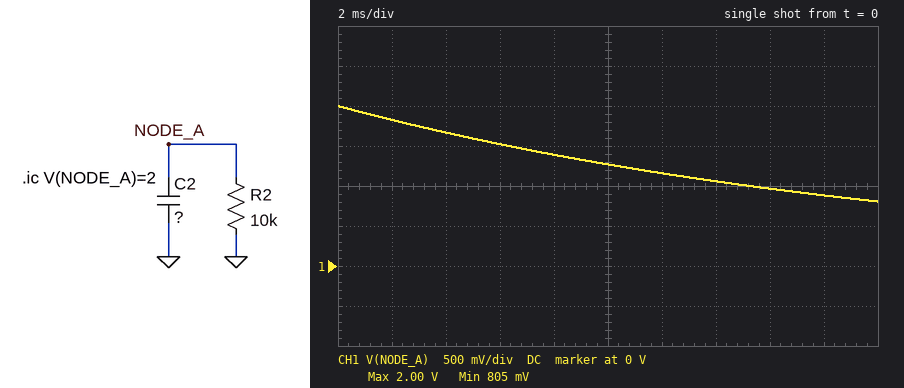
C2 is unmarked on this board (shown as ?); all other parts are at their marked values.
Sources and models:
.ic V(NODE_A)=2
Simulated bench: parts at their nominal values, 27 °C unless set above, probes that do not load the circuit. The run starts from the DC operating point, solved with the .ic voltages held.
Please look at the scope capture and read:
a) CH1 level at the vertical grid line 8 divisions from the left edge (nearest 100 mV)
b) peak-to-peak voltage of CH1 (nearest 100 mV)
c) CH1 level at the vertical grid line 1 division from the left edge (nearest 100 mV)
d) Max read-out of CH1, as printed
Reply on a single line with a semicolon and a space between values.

1.0 V; 1.2 V; 1.8 V; 2.00 V
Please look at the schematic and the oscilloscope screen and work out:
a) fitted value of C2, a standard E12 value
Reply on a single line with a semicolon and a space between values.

2.2 µF
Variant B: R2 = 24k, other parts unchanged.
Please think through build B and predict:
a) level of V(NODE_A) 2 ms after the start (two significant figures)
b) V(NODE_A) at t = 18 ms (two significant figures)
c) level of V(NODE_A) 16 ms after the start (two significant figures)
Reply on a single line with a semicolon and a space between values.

1.9 V; 1.4 V; 1.5 V
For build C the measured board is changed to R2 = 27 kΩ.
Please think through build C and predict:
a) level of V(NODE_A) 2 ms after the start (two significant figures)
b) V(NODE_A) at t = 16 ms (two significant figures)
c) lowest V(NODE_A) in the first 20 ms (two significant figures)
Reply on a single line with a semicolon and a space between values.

1.9 V; 1.5 V; 1.4 V
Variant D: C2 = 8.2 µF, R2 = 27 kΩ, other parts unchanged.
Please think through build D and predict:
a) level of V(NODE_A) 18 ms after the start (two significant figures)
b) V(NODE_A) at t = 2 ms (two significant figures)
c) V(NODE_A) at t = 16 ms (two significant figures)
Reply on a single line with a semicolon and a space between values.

1.8 V; 2.0 V; 1.9 V
